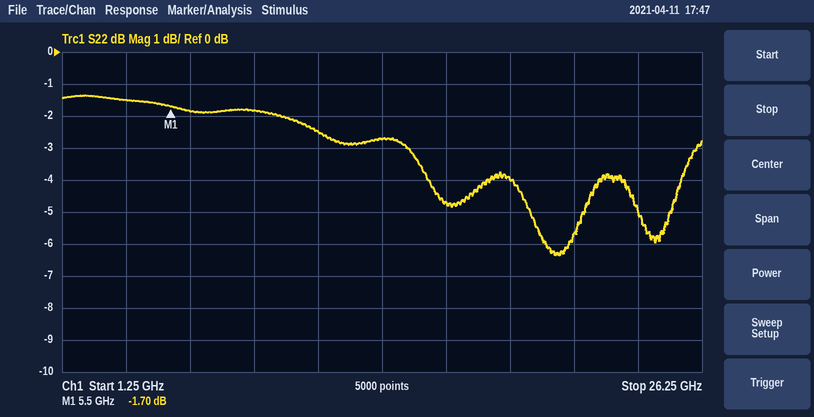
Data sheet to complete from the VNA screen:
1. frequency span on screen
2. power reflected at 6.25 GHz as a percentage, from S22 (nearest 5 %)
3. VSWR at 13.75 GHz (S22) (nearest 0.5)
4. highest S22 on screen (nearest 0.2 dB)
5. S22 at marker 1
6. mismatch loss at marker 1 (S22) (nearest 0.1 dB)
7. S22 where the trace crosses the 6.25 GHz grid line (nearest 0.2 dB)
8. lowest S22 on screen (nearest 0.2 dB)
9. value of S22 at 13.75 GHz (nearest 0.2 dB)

25 GHz
65 %
6.5
-1.4 dB
-1.70 dB
4.9 dB
-1.8 dB
-6.4 dB
-2.8 dB
